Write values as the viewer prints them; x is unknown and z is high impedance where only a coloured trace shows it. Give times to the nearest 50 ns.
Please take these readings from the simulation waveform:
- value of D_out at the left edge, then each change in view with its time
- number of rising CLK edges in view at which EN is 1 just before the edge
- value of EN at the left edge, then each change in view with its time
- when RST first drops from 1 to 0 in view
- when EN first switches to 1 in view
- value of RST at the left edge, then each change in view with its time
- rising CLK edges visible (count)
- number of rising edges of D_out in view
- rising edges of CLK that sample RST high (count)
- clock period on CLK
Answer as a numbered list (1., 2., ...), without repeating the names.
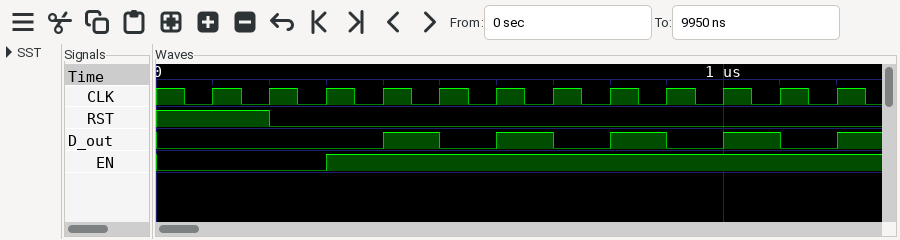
1. 0, 1 at 400 ns, 0 at 500 ns, 1 at 600 ns, 0 at 700 ns, 1 at 800 ns, 0 at 900 ns, 1 at 1000 ns, 0 at 1100 ns, 1 at 1200 ns
2. 9
3. 0, 1 at 300 ns
4. 200 ns
5. 300 ns
6. 1, 0 at 200 ns
7. 12
8. 5
9. 2
10. 100 ns
